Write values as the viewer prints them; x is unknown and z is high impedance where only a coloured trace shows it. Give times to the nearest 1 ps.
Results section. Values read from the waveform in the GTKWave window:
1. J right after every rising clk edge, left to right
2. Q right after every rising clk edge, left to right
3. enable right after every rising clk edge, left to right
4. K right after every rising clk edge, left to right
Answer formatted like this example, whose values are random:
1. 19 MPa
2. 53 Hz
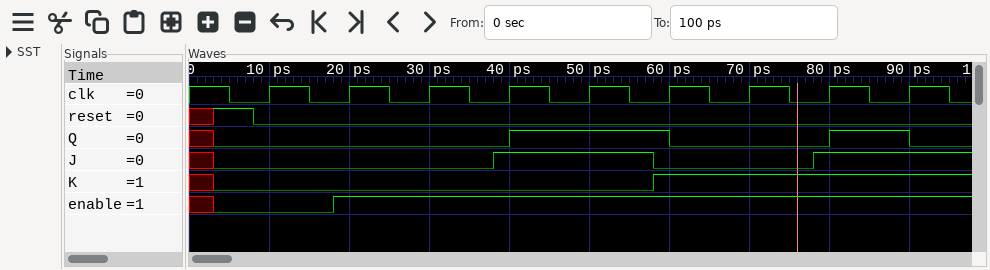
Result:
1. 0 0 0 1 1 0 0 1 1
2. 0 0 0 1 1 0 0 1 0
3. 0 1 1 1 1 1 1 1 1
4. 0 0 0 0 0 1 1 1 1
